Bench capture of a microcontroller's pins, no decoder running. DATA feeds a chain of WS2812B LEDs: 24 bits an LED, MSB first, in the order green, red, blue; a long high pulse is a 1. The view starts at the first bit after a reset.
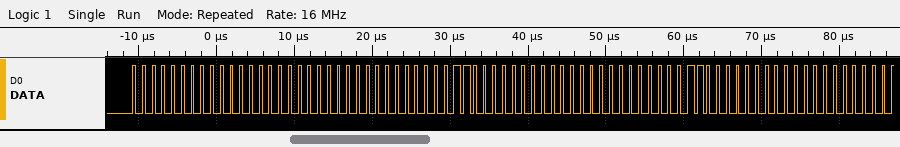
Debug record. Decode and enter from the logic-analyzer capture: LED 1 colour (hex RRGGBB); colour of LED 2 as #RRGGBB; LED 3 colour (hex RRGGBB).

#000000
#600000
#600000
